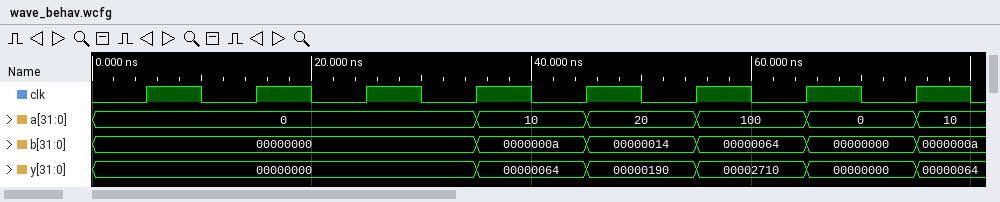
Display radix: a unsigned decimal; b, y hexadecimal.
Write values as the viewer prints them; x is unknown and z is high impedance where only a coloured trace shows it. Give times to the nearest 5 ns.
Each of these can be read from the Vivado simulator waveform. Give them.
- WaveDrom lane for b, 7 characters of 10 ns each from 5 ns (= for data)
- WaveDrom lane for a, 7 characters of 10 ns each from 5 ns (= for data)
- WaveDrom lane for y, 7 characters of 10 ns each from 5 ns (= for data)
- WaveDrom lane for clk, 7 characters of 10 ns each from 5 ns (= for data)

{name: 'b', wave: '=..====', data: '00000000 0000000a 00000014 00000064 00000000'}
{name: 'a', wave: '=..====', data: '0 10 20 100 0'}
{name: 'y', wave: '=..====', data: '00000000 00000064 00000190 00002710 00000000'}
{name: 'clk', wave: 'p......'}
